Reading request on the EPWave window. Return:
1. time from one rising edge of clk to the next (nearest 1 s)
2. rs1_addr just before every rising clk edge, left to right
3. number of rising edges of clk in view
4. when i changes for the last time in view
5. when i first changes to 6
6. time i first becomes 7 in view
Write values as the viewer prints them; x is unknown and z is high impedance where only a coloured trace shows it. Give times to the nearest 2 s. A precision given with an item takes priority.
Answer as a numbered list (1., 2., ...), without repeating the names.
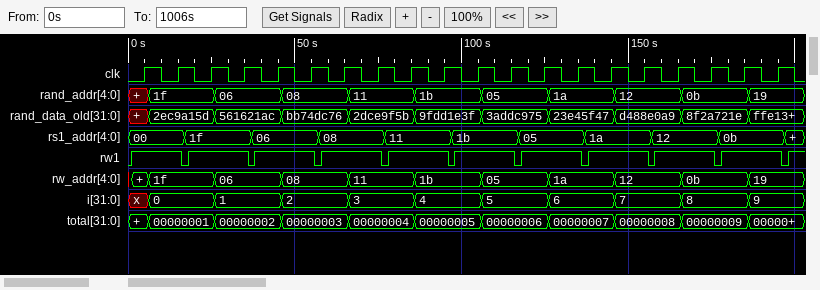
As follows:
1. 10 s
2. 00, 00, 1f, 1f, 06, 06, 08, 08, 11, 11, 1b, 1b, 05, 05, 1a, 1a, 12, 12, 0b, 0b
3. 20
4. 186 s
5. 126 s
6. 146 s
